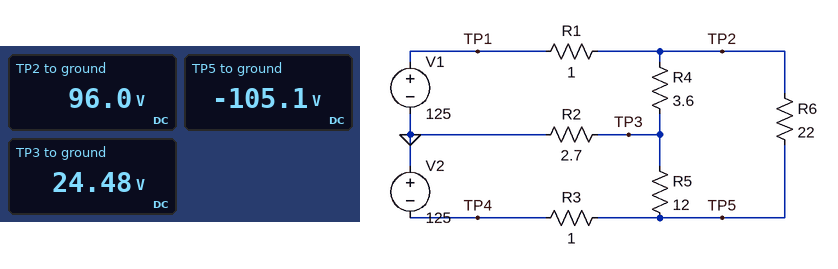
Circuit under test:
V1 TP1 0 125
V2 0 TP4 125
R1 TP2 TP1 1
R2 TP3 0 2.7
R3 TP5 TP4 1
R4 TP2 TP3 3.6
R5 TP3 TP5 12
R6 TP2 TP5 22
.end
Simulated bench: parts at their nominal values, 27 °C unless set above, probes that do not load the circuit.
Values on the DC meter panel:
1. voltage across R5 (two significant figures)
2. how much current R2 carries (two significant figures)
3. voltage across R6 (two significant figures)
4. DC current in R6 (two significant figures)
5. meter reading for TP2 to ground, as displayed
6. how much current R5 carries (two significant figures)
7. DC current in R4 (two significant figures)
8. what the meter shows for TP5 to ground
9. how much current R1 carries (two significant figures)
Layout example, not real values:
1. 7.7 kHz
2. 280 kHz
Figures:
1. 130 V
2. 9.1 A
3. 200 V
4. 9.1 A
5. 96.0 V
6. 11 A
7. 20 A
8. -105.1 V
9. 29 A
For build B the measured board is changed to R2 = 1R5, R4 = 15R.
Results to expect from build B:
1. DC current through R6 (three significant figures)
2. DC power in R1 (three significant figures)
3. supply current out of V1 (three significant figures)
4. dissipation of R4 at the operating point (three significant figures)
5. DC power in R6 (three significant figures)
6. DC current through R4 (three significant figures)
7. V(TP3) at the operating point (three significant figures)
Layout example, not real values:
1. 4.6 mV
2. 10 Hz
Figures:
1. 9.75 A
2. 292 W
3. 17.1 A
4. 806 W
5. 2.09 kW
6. 7.33 A
7. -2.06 V
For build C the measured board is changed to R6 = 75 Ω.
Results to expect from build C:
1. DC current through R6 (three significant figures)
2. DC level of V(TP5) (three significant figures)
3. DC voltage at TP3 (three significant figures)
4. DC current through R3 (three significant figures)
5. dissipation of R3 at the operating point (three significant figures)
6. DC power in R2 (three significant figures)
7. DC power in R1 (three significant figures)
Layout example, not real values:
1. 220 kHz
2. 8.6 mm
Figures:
1. 2.83 A
2. -111 V
3. 25.8 V
4. 14.2 A
5. 202 W
6. 247 W
7. 565 W
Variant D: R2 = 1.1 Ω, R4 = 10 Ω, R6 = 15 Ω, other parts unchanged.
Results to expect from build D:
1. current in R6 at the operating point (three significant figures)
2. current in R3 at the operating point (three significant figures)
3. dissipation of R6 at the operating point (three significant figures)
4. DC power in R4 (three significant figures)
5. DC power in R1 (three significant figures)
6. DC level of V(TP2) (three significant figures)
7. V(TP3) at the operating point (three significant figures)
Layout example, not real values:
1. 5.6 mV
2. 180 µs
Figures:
1. 13.6 A
2. 22.3 A
3. 2.78 kW
4. 999 W
5. 557 W
6. 101 V
7. 1.45 V
